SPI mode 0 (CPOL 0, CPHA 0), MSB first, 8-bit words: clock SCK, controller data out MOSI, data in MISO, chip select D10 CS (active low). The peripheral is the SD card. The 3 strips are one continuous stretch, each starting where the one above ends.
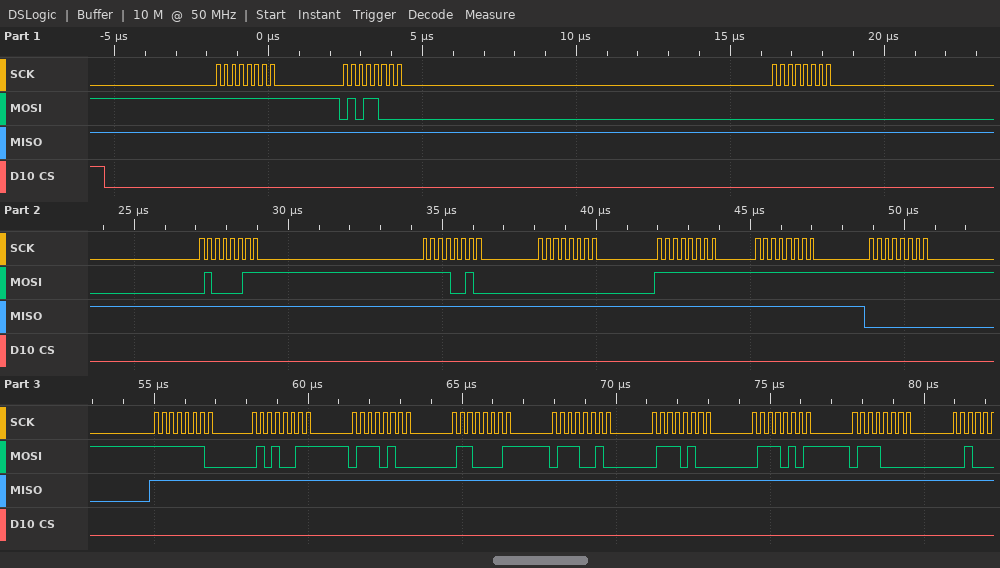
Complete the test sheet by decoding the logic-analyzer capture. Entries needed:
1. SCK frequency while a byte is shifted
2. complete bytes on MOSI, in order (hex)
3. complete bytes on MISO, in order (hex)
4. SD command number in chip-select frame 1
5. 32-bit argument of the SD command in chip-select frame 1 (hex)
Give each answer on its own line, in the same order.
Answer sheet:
4 MHz
FF 58 00 43 F2 00 FF FF FF FE 53 74 61 72 74 75 70
FF FF FF FF FF FF FF FF 00 FF FF FF FF FF FF FF FF
CMD24
0x0043F200
